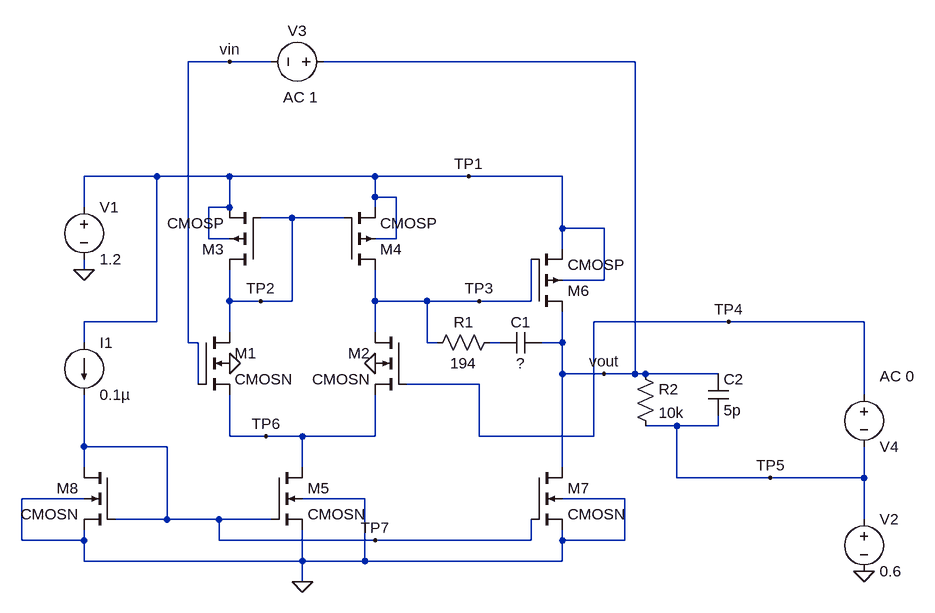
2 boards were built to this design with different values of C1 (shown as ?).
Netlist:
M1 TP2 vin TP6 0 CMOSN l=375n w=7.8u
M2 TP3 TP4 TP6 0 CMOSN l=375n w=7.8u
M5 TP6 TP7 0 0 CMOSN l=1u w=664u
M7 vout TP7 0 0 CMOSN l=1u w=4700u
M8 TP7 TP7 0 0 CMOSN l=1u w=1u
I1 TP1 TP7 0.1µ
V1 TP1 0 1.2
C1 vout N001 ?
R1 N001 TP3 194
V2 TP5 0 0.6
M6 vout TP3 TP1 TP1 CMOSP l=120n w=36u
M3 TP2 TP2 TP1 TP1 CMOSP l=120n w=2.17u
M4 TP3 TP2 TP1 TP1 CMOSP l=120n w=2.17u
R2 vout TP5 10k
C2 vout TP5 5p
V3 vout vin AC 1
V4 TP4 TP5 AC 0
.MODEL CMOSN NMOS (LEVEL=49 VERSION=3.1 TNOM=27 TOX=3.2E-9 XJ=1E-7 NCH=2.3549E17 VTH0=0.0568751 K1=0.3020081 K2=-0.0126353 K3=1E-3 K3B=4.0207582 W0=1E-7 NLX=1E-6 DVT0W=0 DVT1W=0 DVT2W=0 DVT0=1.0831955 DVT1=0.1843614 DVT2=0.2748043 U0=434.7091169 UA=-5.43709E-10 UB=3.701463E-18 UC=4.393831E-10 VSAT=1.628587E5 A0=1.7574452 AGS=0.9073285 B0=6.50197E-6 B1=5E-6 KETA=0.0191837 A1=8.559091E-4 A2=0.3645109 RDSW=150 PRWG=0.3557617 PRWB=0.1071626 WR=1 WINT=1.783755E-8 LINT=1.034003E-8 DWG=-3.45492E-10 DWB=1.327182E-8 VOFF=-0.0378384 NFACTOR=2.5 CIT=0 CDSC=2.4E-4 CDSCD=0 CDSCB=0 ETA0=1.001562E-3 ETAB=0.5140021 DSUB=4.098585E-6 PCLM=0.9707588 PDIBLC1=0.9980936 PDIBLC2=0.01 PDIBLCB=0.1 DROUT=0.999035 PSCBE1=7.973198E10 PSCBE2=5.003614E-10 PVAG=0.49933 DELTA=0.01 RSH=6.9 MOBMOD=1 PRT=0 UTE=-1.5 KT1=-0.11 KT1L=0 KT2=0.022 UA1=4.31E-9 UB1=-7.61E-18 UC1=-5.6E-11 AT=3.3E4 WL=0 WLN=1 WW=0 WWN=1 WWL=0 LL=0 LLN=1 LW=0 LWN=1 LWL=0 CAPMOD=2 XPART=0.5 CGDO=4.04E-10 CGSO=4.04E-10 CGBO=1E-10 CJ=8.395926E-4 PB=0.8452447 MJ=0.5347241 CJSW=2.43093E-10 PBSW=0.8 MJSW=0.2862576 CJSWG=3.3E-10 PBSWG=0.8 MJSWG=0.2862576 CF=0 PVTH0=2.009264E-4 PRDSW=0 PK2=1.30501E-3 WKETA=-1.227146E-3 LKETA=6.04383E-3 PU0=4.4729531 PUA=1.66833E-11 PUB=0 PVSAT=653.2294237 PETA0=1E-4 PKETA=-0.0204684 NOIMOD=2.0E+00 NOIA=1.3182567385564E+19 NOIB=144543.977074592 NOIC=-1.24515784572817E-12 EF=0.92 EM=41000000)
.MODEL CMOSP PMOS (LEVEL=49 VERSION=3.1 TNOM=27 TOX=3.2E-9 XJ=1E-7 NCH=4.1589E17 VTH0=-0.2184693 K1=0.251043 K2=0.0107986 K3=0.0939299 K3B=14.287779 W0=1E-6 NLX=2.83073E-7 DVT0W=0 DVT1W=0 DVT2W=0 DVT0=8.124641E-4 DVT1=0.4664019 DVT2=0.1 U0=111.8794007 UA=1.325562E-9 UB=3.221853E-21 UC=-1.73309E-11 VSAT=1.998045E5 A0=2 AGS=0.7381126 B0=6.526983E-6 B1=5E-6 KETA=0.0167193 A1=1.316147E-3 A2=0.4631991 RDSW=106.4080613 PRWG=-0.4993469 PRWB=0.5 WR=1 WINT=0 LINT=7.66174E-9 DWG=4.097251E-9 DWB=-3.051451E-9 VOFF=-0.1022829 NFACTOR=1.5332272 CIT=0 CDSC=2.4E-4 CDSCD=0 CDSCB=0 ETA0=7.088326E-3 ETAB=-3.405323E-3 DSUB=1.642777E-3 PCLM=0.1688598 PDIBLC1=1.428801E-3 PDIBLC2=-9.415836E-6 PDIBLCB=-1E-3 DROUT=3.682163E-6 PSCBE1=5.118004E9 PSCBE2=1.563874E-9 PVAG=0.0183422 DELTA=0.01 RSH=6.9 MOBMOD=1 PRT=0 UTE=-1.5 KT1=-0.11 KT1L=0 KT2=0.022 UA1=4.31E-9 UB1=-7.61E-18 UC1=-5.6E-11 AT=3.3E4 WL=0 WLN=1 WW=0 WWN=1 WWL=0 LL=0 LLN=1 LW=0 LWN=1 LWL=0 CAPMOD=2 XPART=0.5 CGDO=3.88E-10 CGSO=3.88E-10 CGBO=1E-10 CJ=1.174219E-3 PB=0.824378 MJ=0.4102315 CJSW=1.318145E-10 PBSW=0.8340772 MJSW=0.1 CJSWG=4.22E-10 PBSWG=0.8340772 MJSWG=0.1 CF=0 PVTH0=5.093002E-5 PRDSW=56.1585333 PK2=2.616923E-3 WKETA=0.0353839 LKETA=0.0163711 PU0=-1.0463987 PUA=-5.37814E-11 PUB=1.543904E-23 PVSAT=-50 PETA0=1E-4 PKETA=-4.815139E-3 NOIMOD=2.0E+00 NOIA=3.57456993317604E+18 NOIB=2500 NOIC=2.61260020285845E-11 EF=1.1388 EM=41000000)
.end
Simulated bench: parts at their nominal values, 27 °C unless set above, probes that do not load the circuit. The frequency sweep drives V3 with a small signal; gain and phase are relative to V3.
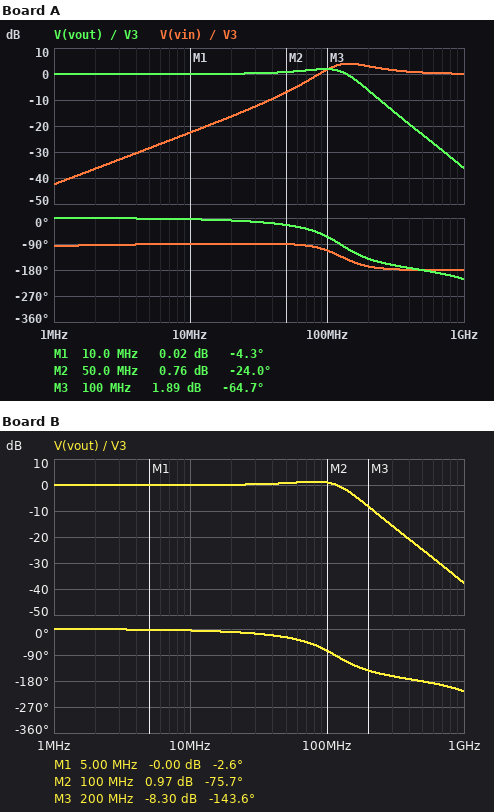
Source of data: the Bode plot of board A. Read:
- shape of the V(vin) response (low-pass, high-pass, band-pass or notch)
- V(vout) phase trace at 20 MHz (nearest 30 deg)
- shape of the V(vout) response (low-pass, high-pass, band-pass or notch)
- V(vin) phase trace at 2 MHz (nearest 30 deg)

high-pass
0 deg
low-pass
-90 deg
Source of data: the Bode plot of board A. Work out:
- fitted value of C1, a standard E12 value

680 fF
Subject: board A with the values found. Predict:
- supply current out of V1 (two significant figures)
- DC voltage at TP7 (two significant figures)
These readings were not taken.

610 µA
190 mV
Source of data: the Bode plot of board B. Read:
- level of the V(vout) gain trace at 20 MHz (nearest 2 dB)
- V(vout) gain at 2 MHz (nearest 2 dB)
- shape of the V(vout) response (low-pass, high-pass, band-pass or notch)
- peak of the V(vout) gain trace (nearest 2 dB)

0 dB
0 dB
low-pass
2 dB
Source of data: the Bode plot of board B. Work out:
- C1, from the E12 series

820 fF
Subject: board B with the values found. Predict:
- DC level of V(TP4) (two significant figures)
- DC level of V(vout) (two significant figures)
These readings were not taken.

600 mV
600 mV
